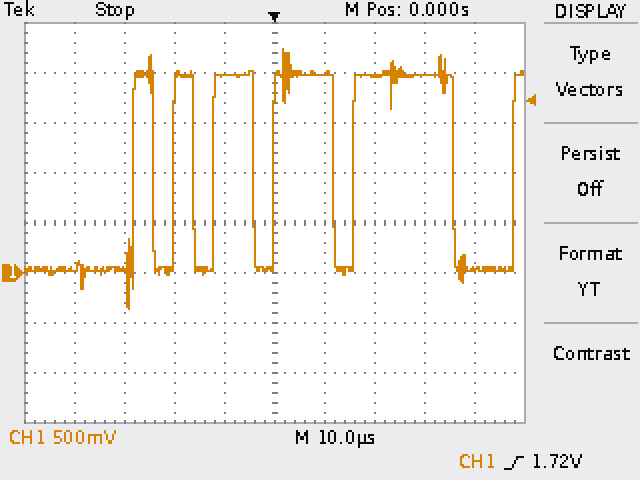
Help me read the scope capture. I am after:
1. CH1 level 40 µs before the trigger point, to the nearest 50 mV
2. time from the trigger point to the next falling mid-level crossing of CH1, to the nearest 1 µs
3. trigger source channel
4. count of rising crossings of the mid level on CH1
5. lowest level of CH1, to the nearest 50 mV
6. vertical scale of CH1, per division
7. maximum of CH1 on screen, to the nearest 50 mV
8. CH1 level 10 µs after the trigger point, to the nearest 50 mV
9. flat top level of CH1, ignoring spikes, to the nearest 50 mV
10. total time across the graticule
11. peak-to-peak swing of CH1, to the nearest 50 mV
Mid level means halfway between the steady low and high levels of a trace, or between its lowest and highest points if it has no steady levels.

50 mV
12 µs
CH1
6
-350 mV
500 mV
2.25 V
2.00 V
2.00 V
100 µs
2.60 V
